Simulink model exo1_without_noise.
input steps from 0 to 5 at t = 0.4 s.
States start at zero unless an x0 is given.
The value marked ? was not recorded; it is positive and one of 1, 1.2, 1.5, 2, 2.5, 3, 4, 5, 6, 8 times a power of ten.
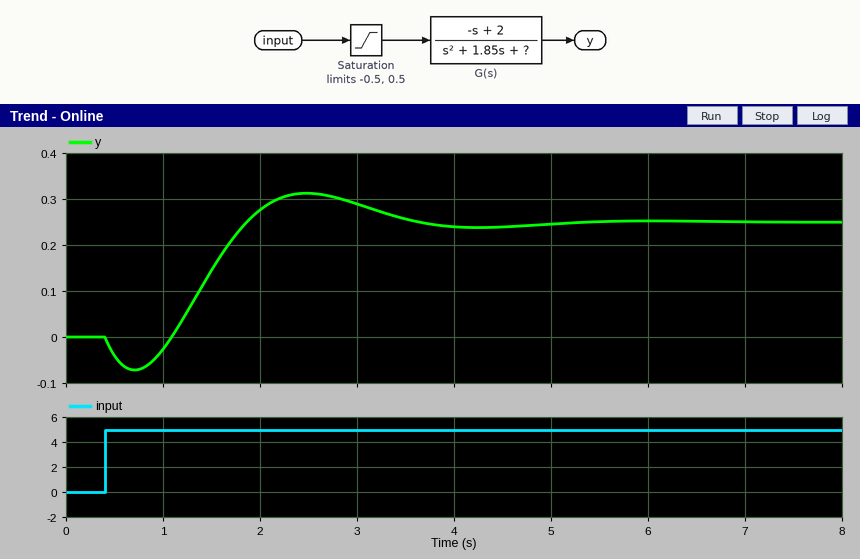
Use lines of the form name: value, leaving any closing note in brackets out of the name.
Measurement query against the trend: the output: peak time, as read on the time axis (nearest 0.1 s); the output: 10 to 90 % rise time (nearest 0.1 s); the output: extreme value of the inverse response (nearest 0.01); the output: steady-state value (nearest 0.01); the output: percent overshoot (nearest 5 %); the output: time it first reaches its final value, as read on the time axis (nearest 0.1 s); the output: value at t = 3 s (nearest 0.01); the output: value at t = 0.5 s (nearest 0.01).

the output: peak time, as read on the time axis: 2.5 s
the output: 10 to 90 % rise time: 0.6 s
the output: extreme value of the inverse response: -0.07
the output: steady-state value: 0.25
the output: percent overshoot: 25 %
the output: time it first reaches its final value, as read on the time axis: 1.9 s
the output: value at t = 3 s: 0.29
the output: value at t = 0.5 s: -0.04
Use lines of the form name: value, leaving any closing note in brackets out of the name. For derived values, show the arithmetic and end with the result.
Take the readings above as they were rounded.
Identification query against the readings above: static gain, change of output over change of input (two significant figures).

static gain, change of output over change of input: (0.25 - 0) / (5 - 0) = 0.050
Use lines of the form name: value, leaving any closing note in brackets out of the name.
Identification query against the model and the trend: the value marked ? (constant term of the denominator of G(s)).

the value marked ? (constant term of the denominator of G(s)): 4
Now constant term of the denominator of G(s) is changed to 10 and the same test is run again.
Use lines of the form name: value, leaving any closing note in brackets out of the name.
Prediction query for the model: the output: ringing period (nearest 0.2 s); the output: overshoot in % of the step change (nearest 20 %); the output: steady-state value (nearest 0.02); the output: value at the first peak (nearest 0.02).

the output: ringing period: 2.0 s
the output: overshoot in % of the step change: 60 %
the output: steady-state value: 0.10
the output: value at the first peak: 0.16
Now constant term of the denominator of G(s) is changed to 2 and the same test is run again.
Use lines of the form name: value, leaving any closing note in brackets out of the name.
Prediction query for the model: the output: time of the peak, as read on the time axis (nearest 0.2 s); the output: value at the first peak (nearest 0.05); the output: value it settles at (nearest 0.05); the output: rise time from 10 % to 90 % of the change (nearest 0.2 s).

the output: time of the peak, as read on the time axis: 3.6 s
the output: value at the first peak: 0.55
the output: value it settles at: 0.50
the output: rise time from 10 % to 90 % of the change: 1.2 s
